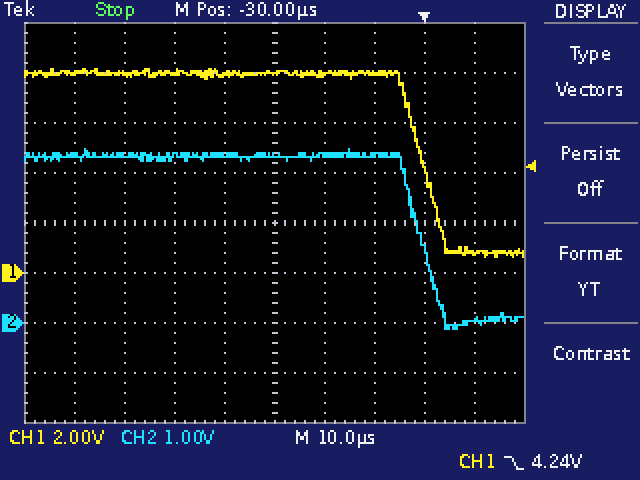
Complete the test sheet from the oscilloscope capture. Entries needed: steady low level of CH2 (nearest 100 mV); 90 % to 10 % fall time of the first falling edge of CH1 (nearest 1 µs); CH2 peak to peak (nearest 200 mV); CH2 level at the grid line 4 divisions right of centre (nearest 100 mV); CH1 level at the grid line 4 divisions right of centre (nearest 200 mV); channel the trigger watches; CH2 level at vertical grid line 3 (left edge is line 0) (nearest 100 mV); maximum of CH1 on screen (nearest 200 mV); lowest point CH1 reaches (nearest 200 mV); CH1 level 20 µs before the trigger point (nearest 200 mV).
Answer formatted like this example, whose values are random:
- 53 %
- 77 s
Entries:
- 100 mV
- 8 µs
- 3.6 V
- 100 mV
- 800 mV
- CH1
- 3.3 V
- 8.2 V
- 600 mV
- 8.0 V
